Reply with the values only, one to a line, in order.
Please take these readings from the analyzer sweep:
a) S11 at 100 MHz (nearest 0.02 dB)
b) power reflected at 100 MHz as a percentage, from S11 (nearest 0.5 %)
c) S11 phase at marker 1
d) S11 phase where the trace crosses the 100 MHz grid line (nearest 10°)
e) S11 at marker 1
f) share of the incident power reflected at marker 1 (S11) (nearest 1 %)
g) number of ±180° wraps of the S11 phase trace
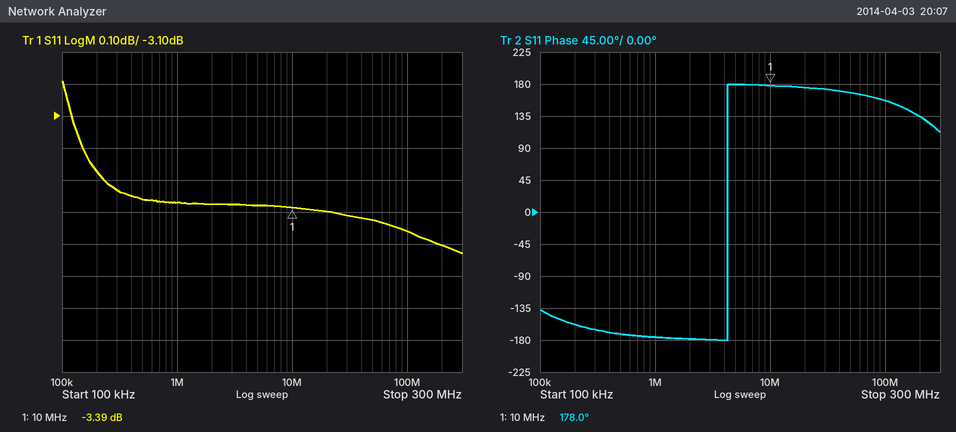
-3.46 dB
45.0 %
178.0°
160°
-3.39 dB
46 %
1
